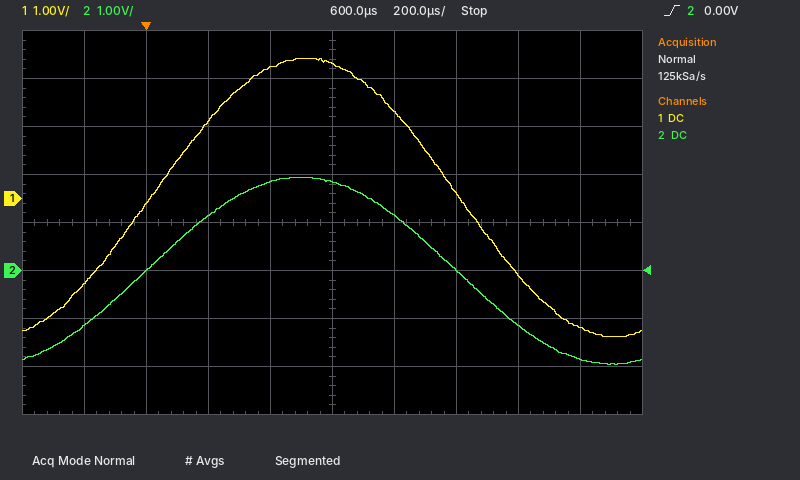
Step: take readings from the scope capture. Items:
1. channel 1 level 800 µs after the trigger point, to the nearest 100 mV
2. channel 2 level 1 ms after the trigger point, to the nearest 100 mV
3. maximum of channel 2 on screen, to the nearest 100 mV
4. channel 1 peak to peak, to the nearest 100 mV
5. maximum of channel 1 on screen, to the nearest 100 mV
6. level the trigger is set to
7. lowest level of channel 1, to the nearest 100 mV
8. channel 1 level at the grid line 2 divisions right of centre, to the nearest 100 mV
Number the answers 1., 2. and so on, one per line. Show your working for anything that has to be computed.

1. 1.8 V
2. 0.0 V
3. 1.9 V
4. 2.9 V − (-2.9 V) = 5.8 V
5. 2.9 V
6. 0.00 V
7. -2.9 V
8. 100 mV
